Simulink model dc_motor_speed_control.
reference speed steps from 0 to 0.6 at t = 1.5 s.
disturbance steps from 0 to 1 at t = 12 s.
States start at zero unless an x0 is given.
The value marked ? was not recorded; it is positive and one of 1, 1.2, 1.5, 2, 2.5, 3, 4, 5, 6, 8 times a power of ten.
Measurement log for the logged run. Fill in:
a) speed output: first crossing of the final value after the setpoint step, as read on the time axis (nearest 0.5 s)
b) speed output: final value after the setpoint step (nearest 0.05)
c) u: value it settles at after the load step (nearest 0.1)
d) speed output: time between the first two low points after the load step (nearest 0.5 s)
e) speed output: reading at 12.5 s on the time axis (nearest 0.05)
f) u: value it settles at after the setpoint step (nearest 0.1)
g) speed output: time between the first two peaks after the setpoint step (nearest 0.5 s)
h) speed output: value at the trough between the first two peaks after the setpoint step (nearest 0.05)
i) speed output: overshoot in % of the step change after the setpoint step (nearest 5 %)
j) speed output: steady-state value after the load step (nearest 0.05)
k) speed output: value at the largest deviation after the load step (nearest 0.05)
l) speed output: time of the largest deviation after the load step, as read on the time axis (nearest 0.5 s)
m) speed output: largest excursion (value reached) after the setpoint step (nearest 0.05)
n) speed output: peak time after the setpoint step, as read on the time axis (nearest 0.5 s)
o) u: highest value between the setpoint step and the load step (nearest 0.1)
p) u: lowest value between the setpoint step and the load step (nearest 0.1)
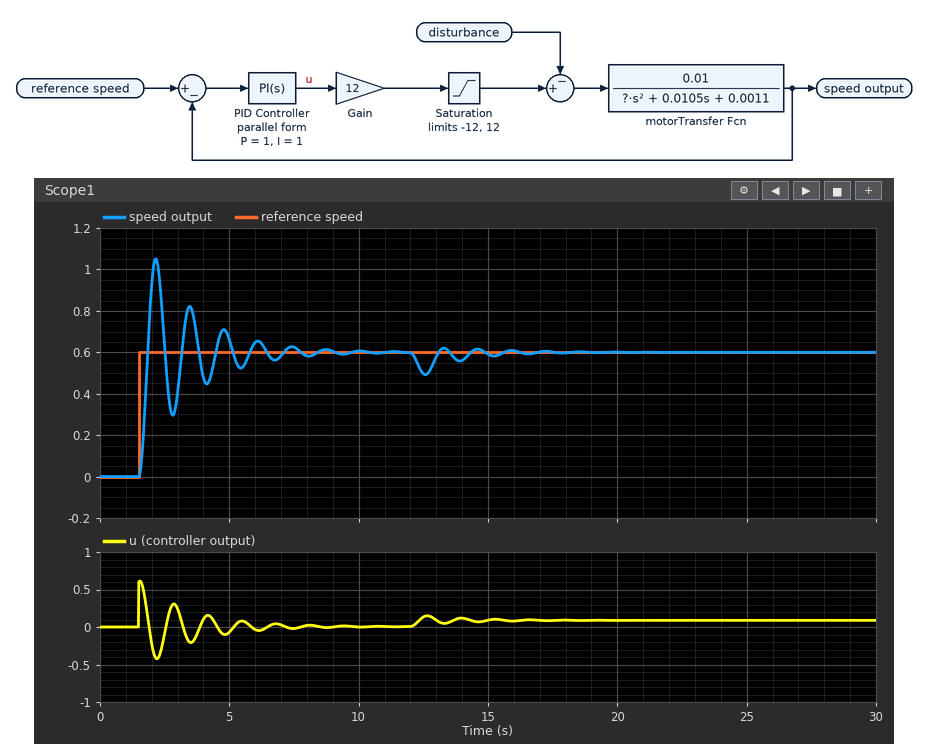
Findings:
2.0 s
0.60
0.1
1.5 s
0.50
0.0
1.5 s
0.30
75 %
0.60
0.50
12.5 s
1.05
2.0 s
0.6
-0.4
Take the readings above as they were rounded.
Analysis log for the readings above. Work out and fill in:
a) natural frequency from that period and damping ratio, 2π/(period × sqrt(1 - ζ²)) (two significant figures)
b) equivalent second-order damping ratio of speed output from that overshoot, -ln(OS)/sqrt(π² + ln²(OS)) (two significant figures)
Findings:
4.2 rad/s
0.091
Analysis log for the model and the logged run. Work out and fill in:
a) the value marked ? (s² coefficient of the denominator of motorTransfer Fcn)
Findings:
0.005
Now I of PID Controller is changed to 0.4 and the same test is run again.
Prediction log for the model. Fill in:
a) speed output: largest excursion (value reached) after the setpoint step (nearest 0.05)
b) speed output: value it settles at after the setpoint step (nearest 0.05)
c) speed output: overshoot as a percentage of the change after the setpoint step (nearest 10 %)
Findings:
0.95
0.60
60 %
